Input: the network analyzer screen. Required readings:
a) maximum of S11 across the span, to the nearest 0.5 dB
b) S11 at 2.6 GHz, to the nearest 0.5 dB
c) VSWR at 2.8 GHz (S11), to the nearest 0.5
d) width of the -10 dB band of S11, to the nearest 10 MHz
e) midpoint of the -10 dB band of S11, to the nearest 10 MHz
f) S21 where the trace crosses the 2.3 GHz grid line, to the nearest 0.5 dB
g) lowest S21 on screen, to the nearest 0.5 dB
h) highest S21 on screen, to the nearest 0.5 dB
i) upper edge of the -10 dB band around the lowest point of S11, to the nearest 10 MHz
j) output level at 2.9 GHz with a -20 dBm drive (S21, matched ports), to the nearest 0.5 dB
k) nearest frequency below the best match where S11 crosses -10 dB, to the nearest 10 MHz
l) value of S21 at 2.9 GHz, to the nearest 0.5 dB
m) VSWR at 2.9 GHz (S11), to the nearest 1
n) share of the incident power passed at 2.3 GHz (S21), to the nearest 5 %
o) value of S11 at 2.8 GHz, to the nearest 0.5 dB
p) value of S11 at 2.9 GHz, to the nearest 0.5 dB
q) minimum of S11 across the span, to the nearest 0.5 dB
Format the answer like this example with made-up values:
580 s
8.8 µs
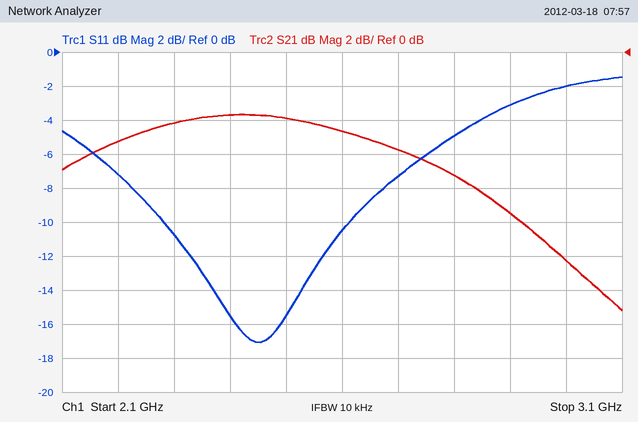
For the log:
-1.5 dB
-10.5 dB
3.5
330 MHz
2.45 GHz
-4.0 dB
-15.0 dB
-3.5 dB
2.61 GHz
-29.5 dBm
2.28 GHz
-9.5 dB
6
40 %
-5.0 dB
-3.0 dB
-17.0 dB
